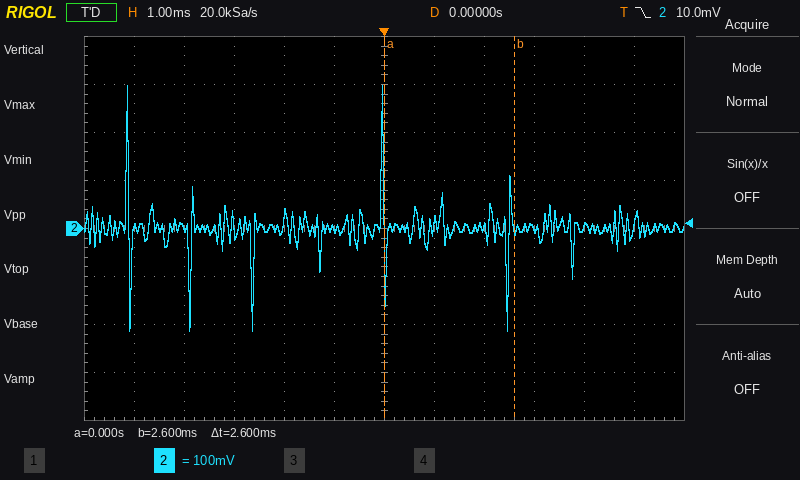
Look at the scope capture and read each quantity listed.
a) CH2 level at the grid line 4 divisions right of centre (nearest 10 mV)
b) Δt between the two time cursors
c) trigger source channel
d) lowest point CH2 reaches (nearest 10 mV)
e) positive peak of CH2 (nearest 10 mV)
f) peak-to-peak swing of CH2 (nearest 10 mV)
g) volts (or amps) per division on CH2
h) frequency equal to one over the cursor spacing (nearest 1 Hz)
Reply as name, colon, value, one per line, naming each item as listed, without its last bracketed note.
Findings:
CH2 level at the grid line 4 divisions right of centre: 0 mV
Δt between the two time cursors: 2.6 ms
trigger source channel: CH2
lowest point CH2 reaches: -210 mV
positive peak of CH2: 300 mV
peak-to-peak swing of CH2: 510 mV
volts (or amps) per division on CH2: 100 mV
frequency equal to one over the cursor spacing: 385 Hz
